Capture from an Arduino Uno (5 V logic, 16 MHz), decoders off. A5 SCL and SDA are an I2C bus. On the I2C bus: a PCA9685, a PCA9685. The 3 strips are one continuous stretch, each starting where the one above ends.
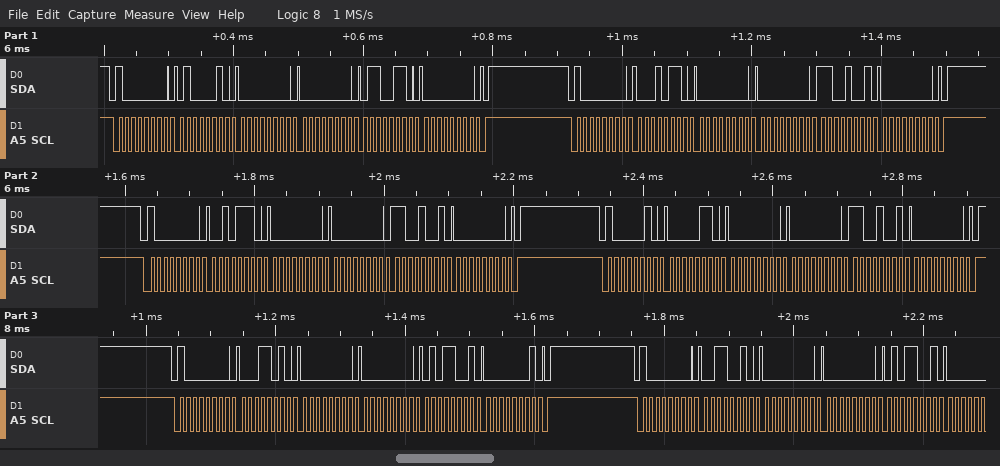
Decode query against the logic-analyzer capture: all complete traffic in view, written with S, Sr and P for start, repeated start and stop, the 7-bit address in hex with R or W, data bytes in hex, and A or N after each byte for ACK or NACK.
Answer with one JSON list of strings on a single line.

["S 40W A 42 A 00 A 00 A 66 A 00 A P S 40W A 16 A 00 A 00 A C9 A 00 A P S 40W A 2E A 00 A 00 A C9 A 00 A P S 41W A 06 A 00 A 00 A C9 A 00 A P S 40W A 1A A 00 A 00 A 59 A 01 A P S 40W A 32 A 00 A 00 A 59 A"]
